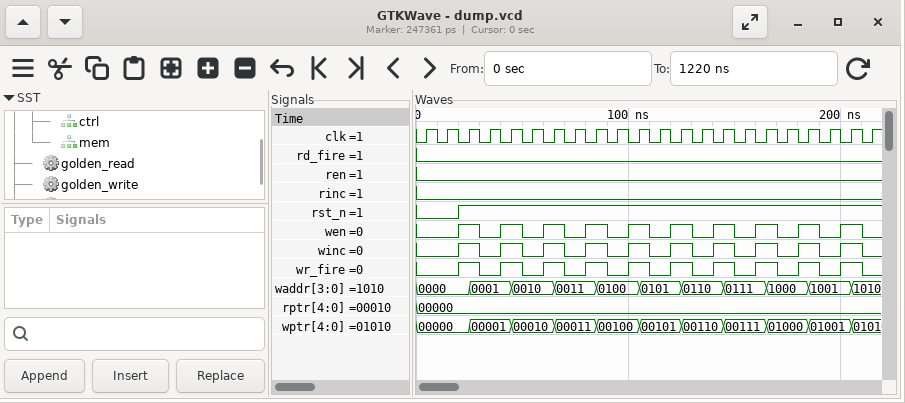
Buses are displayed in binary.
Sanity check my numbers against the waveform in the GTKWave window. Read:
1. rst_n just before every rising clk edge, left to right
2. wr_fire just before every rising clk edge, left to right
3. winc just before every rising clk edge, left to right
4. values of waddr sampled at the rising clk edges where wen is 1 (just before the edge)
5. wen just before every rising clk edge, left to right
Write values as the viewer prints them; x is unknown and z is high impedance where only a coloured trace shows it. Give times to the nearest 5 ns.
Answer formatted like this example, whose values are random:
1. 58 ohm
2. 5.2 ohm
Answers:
1. 0 0 1 1 1 1 1 1 1 1 1 1 1 1 1 1 1 1 1 1 1 1
2. 0 0 1 0 1 0 1 0 1 0 1 0 1 0 1 0 1 0 1 0 1 0
3. 0 0 1 0 1 0 1 0 1 0 1 0 1 0 1 0 1 0 1 0 1 0
4. 0000, 0001, 0010, 0011, 0100, 0101, 0110, 0111, 1000, 1001
5. 0 0 1 0 1 0 1 0 1 0 1 0 1 0 1 0 1 0 1 0 1 0
